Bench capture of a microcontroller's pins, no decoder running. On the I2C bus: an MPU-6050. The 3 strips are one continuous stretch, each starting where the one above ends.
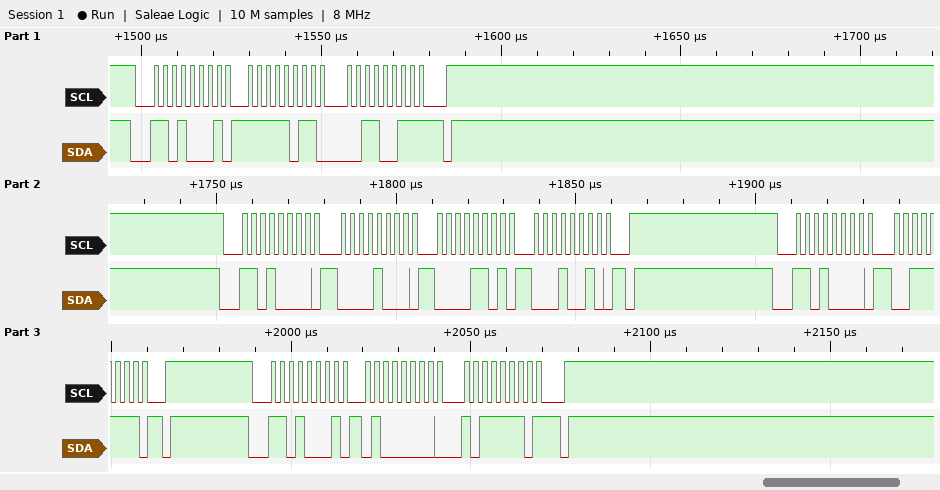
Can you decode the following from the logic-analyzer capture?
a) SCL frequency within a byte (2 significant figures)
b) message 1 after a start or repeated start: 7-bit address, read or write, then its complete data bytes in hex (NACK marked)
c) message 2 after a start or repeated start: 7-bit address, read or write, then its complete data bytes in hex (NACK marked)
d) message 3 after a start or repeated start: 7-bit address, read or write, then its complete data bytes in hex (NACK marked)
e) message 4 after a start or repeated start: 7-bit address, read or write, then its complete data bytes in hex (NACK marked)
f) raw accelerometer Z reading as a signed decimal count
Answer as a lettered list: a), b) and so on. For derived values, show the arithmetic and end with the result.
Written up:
a) 400 kHz
b) 0x68 read: FB 33 NACK
c) 0x68 write: 08 0D 12
d) 0x68 write: 3F
e) 0x68 read: 40 BE NACK
f) 0x40BE = 16574
